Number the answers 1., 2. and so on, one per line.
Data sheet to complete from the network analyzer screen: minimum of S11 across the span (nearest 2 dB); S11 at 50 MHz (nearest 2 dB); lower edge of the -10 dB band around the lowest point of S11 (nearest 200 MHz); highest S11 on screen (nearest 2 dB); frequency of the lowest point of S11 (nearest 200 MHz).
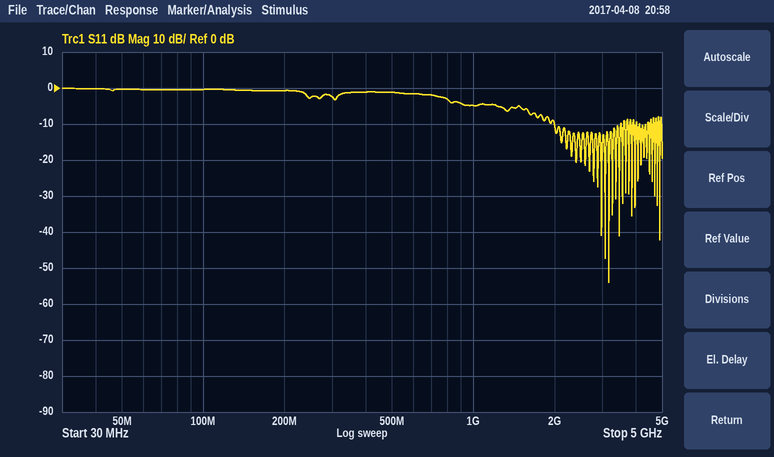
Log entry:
1. -54 dB
2. 0 dB
3. 2.0 GHz
4. 0 dB
5. 3.2 GHz
